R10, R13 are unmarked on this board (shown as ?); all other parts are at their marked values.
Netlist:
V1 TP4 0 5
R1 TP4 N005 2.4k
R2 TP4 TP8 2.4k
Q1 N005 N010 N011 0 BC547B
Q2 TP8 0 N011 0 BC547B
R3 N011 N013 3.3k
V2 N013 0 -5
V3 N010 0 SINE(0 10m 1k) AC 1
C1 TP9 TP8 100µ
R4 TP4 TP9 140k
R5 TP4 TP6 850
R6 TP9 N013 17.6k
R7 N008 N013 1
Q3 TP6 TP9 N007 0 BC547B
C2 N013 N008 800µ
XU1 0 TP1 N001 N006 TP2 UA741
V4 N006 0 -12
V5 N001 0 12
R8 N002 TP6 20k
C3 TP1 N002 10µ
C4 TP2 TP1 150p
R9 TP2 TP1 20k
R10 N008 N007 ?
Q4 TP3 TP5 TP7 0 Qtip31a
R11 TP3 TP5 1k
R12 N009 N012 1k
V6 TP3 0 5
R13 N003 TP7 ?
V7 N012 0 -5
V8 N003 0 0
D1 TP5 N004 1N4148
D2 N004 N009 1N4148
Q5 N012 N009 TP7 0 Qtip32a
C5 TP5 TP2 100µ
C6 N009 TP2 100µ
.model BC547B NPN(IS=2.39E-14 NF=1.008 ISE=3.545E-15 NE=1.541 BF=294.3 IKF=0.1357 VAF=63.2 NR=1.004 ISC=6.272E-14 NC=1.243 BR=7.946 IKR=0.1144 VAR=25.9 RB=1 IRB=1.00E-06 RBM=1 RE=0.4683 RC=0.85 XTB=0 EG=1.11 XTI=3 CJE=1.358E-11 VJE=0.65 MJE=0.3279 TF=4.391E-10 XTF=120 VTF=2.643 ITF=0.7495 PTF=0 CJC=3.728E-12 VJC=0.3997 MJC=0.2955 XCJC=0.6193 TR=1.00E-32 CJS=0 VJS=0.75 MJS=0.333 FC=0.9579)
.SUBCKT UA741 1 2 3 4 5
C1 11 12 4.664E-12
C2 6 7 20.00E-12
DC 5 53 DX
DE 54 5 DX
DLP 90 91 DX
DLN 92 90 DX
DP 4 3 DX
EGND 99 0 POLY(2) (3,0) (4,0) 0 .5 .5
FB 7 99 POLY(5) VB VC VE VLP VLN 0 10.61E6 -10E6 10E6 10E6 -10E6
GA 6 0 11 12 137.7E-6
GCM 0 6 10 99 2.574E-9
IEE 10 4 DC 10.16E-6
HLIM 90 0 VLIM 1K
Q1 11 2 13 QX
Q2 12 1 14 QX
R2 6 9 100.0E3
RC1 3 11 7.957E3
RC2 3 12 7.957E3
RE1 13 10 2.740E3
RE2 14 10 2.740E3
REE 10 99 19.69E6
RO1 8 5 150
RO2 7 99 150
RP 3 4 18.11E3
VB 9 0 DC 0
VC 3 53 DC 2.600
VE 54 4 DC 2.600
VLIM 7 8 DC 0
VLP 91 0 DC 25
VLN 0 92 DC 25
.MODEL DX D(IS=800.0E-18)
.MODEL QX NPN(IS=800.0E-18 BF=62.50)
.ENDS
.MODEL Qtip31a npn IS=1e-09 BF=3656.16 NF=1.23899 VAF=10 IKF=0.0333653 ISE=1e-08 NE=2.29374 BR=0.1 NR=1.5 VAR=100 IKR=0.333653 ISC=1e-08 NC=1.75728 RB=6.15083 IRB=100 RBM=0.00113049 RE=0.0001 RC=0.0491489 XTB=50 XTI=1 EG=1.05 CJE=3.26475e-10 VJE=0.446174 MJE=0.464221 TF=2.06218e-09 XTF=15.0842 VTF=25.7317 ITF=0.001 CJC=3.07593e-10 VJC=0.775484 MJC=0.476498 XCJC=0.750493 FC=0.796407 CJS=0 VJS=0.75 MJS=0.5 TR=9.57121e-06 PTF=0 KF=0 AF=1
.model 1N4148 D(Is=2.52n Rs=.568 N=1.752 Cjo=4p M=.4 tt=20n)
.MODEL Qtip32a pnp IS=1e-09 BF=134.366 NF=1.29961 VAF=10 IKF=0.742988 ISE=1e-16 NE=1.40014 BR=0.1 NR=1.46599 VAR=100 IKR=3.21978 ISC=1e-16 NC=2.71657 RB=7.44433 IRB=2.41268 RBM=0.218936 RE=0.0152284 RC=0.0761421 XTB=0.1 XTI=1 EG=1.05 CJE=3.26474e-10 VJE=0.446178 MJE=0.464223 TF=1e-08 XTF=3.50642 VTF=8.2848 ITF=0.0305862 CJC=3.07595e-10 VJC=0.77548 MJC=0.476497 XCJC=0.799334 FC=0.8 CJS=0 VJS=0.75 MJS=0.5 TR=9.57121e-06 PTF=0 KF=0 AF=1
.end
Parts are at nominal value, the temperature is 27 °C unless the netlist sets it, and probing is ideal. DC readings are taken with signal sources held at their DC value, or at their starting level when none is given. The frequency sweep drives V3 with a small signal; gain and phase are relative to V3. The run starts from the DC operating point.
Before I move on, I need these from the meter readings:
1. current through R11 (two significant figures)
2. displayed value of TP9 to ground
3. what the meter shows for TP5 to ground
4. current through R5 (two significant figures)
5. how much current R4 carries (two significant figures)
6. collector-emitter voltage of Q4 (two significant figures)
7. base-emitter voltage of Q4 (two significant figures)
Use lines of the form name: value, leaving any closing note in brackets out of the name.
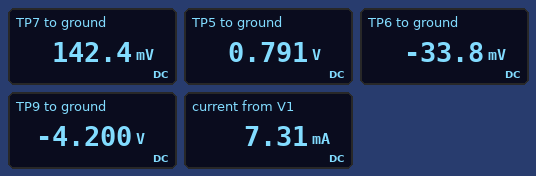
current through R11: 4.2 mA
displayed value of TP9 to ground: -4.200 V
what the meter shows for TP5 to ground: 0.791 V
current through R5: 5.9 mA
how much current R4 carries: 66 µA
collector-emitter voltage of Q4: 4.9 V
base-emitter voltage of Q4: 650 mV
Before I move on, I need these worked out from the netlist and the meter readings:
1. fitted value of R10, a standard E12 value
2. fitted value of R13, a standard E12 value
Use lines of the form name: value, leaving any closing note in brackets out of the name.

fitted value of R10, a standard E12 value: 18 Ω
fitted value of R13, a standard E12 value: 27 Ω
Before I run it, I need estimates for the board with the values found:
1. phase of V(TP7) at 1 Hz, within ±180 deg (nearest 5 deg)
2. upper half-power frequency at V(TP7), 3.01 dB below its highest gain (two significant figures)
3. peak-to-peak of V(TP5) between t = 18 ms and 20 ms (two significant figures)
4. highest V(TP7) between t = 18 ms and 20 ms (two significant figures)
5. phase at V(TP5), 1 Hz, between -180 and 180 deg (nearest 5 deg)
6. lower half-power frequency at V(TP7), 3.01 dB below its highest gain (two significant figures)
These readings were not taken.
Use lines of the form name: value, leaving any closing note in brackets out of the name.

phase of V(TP7) at 1 Hz, within ±180 deg: 110 deg
upper half-power frequency at V(TP7), 3.01 dB below its highest gain: 50 kHz
peak-to-peak of V(TP5) between t = 18 ms and 20 ms: 9.3 V
highest V(TP7) between t = 18 ms and 20 ms: 4.7 V
phase at V(TP5), 1 Hz, between -180 and 180 deg: 110 deg
lower half-power frequency at V(TP7), 3.01 dB below its highest gain: 2.3 Hz
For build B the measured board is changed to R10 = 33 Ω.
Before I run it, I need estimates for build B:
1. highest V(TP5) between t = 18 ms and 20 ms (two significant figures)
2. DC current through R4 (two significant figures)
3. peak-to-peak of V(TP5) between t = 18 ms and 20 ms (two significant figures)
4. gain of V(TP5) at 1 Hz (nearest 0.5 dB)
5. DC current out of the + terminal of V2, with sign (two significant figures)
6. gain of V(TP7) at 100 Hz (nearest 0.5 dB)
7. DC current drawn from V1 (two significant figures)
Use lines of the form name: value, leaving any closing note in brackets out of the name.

highest V(TP5) between t = 18 ms and 20 ms: 5.1 V
DC current through R4: 65 µA
peak-to-peak of V(TP5) between t = 18 ms and 20 ms: 8.1 V
gain of V(TP5) at 1 Hz: 44.0 dB
DC current out of the + terminal of V2, with sign: -6.4 mA
gain of V(TP7) at 100 Hz: 52.5 dB
DC current drawn from V1: 6.4 mA
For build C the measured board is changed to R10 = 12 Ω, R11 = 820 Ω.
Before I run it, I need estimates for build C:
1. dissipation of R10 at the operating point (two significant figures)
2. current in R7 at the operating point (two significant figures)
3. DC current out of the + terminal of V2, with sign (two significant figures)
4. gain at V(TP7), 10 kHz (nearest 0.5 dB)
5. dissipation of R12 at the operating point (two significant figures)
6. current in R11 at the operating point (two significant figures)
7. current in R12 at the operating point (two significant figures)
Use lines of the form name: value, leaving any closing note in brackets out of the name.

dissipation of R10 at the operating point: 490 µW
current in R7 at the operating point: 6.4 mA
DC current out of the + terminal of V2, with sign: -7.8 mA
gain at V(TP7), 10 kHz: 58.0 dB
dissipation of R12 at the operating point: 24 mW
current in R11 at the operating point: 4.7 mA
current in R12 at the operating point: 4.9 mA
